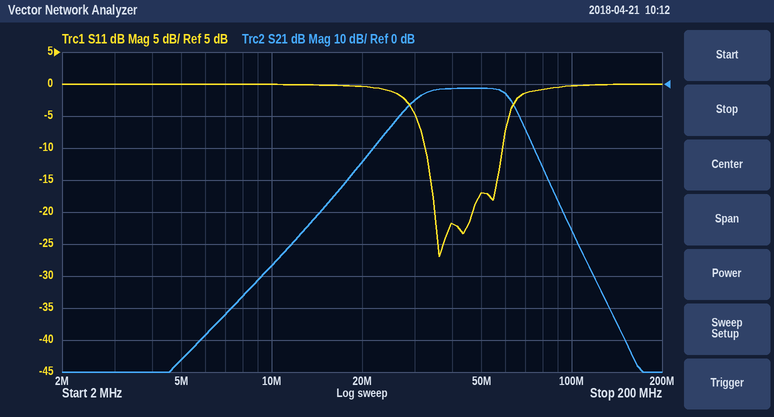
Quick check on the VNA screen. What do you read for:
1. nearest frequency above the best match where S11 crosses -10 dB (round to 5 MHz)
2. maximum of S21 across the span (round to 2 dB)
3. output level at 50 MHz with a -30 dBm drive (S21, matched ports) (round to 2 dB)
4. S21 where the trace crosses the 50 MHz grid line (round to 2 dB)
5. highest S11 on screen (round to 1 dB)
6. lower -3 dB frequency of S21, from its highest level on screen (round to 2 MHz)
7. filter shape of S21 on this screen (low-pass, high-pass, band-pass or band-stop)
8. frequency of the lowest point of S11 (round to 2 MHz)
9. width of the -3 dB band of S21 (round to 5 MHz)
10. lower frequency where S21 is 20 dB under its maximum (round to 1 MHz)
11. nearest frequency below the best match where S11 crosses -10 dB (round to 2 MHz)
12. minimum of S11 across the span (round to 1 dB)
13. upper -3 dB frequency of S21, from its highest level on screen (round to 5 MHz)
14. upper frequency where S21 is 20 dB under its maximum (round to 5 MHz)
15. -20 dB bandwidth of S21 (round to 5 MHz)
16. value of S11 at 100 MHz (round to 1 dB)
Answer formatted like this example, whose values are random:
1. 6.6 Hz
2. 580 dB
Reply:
1. 60 MHz
2. -2 dB
3. -32 dBm
4. -2 dB
5. 0 dB
6. 30 MHz
7. band-pass
8. 36 MHz
9. 30 MHz
10. 21 MHz
11. 32 MHz
12. -27 dB
13. 60 MHz
14. 75 MHz
15. 55 MHz
16. 0 dB
